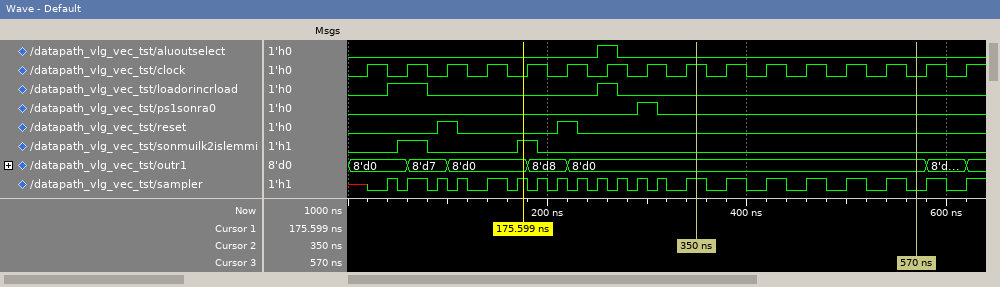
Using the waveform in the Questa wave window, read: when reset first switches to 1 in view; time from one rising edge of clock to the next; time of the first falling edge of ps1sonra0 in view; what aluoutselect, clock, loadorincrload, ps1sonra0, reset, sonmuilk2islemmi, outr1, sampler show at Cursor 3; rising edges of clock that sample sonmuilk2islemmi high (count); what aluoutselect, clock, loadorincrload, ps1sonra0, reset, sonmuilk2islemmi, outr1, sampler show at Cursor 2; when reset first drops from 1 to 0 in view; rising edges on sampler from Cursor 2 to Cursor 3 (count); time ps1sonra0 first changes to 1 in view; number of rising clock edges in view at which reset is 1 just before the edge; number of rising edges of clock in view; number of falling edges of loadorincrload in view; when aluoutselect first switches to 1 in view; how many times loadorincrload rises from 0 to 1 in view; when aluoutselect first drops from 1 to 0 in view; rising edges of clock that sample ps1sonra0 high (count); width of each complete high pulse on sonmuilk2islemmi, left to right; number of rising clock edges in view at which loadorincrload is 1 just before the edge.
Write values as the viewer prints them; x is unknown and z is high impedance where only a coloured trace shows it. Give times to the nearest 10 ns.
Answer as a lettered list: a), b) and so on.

a) 90 ns
b) 40 ns
c) 310 ns
d) aluoutselect=0, clock=0, loadorincrload=0, ps1sonra0=0, reset=0, sonmuilk2islemmi=0, outr1=8'd0, sampler=0
e) 2
f) aluoutselect=0, clock=1, loadorincrload=0, ps1sonra0=0, reset=0, sonmuilk2islemmi=0, outr1=8'd0, sampler=1
g) 110 ns
h) 5
i) 290 ns
j) 2
k) 16
l) 2
m) 250 ns
n) 2
o) 270 ns
p) 1
q) 30 ns, 20 ns
r) 2
